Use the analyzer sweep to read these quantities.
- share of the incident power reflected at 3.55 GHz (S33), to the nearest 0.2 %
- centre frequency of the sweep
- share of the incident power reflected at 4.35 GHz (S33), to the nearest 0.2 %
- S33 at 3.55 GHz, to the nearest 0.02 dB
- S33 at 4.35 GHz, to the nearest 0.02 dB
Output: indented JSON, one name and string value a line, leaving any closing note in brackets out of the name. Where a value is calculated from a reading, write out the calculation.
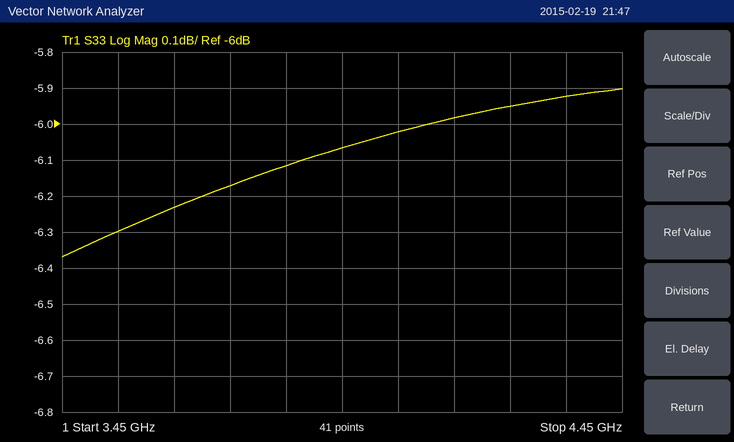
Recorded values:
{
  "share of the incident power reflected at 3.55 GHz (S33), to the nearest 0.2 %": "10^(-6.3/10) ≈ 23.4 %",
  "centre frequency of the sweep": "3.95 GHz",
  "share of the incident power reflected at 4.35 GHz (S33), to the nearest 0.2 %": "10^(-5.92/10) ≈ 25.6 %",
  "S33 at 3.55 GHz, to the nearest 0.02 dB": "-6.30 dB",
  "S33 at 4.35 GHz, to the nearest 0.02 dB": "-5.92 dB"
}
